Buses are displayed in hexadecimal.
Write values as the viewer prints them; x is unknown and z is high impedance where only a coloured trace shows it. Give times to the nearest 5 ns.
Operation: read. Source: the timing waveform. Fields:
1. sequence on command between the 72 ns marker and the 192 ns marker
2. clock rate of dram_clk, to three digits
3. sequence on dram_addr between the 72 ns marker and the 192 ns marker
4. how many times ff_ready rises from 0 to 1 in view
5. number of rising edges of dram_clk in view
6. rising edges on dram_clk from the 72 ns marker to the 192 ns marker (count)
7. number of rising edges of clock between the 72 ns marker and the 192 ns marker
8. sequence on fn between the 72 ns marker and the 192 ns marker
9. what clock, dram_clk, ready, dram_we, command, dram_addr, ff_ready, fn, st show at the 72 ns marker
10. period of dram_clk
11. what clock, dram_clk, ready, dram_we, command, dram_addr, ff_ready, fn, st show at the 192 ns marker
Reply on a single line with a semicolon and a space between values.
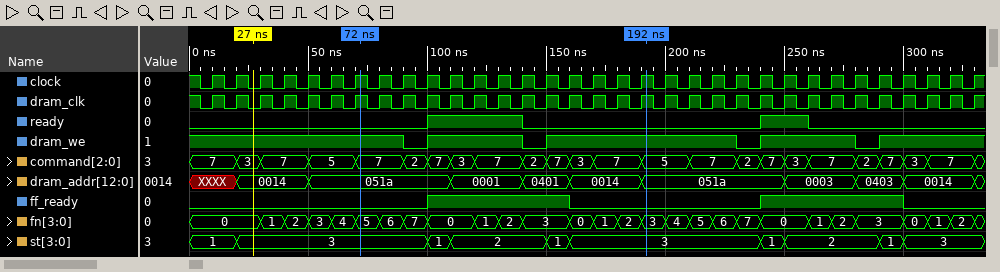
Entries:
7, 2, 7, 3, 7, 2, 7, 3, 7, 5; 100 MHz; 051a, 0001, 0401, 0014, 051a; 2; 33; 12; 12; 5, 6, 7, 0, 1, 2, 3, 0, 1, 2, 3; clock=1, dram_clk=1, ready=0, dram_we=1, command=7, dram_addr=051a, ff_ready=0, fn=5, st=3; 10 ns; clock=1, dram_clk=1, ready=0, dram_we=1, command=5, dram_addr=051a, ff_ready=0, fn=3, st=3
